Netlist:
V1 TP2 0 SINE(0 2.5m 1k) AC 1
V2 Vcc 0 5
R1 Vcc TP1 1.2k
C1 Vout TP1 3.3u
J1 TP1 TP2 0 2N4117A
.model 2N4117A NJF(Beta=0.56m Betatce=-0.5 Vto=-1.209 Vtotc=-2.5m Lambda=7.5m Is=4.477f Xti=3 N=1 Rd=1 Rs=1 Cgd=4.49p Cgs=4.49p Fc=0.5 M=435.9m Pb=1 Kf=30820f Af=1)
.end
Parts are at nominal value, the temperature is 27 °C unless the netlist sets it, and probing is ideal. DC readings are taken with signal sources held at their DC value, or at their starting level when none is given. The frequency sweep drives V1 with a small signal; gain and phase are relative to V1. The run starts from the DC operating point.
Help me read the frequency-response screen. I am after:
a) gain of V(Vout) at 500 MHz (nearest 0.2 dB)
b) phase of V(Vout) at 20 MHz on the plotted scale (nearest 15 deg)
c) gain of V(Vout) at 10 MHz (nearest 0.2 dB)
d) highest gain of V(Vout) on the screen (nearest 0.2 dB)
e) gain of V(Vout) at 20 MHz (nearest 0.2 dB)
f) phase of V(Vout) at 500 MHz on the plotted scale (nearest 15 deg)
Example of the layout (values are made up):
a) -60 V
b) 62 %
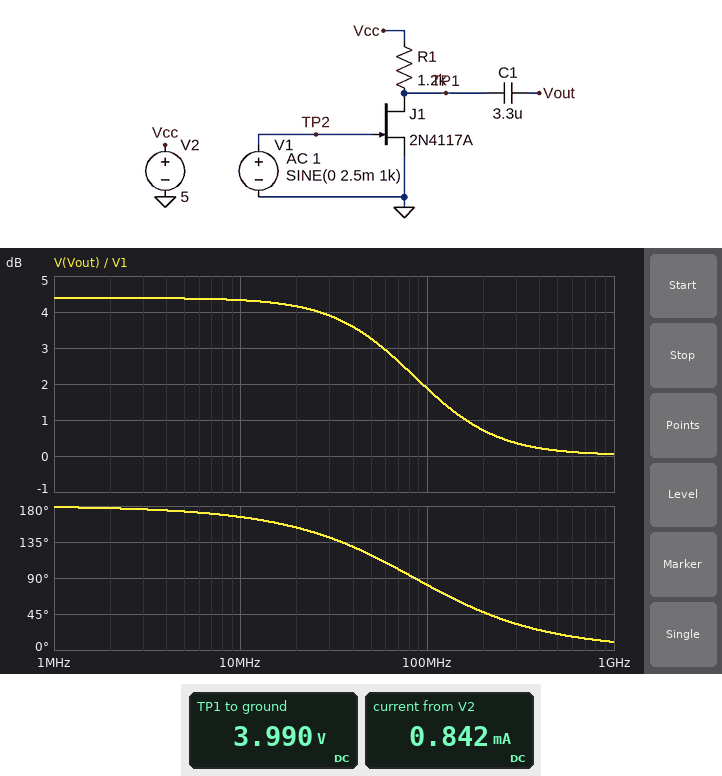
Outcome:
a) 0.2 dB
b) 150 deg
c) 4.4 dB
d) 4.4 dB
e) 4.2 dB
f) 15 deg
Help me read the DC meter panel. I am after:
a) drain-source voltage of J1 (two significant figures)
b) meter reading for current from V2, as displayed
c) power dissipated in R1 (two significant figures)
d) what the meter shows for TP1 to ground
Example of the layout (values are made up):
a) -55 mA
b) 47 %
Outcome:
a) 4.0 V
b) 0.842 mA
c) 850 µW
d) 3.990 V
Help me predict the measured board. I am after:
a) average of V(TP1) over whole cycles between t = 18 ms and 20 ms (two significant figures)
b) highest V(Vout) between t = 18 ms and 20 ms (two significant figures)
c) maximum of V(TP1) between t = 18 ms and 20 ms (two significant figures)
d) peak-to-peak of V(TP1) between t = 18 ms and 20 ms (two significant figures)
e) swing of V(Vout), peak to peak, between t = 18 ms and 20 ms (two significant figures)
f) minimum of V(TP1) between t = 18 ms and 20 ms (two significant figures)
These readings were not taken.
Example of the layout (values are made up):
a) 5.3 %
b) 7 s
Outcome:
a) 4.0 V
b) 4.1 mV
c) 4.0 V
d) 8.3 mV
e) 8.3 mV
f) 4.0 V
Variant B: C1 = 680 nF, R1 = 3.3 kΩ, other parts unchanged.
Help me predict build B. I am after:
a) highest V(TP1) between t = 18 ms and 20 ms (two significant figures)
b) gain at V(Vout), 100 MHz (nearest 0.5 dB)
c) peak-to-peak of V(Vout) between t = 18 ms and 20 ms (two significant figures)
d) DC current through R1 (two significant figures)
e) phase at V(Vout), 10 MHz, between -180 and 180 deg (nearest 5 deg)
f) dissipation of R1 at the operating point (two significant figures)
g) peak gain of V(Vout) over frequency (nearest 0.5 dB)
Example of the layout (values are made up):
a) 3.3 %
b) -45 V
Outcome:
a) 2.3 V
b) 2.5 dB
c) 22 mV
d) 830 µA
e) 145 deg
f) 2.3 mW
g) 13.0 dB
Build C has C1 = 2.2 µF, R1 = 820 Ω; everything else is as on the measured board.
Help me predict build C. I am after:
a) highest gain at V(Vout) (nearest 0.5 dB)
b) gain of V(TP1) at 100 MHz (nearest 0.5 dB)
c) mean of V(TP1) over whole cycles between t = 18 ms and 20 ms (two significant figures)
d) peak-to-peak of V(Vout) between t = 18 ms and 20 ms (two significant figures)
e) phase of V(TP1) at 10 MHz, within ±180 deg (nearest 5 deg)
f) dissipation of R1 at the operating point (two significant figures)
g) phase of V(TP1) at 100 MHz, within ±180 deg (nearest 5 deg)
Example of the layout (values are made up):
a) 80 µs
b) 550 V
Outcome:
a) 1.0 dB
b) 0.5 dB
c) 4.3 V
d) 5.7 mV
e) 170 deg
f) 580 µW
g) 95 deg
